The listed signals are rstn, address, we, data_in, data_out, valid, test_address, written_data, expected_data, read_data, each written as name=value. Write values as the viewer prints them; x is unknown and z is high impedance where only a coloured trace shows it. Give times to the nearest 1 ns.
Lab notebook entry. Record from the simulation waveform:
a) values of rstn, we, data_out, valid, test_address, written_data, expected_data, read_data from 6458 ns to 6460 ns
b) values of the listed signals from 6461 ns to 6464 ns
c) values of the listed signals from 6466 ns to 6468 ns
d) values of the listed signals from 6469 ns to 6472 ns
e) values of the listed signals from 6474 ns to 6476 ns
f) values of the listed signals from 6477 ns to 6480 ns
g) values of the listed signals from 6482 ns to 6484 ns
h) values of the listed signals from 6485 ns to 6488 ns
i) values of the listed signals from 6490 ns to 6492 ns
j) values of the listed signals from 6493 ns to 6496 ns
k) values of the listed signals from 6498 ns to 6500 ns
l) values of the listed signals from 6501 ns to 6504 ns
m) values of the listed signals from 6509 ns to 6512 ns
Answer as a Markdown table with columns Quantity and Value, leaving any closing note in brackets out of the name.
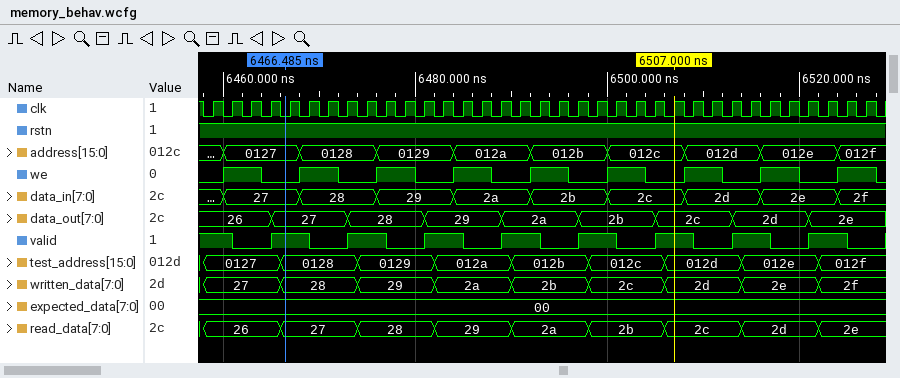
| Quantity | Value |
|---|---|
| values of rstn, we, data_out, valid, test_address, written_data, expected_data, read_data from 6458 ns to 6460 ns | rstn=1, we=0, data_out=26, valid=1, test_address=0127, written_data=27, expected_data=00, read_data=26 |
| values of the listed signals from 6461 ns to 6464 ns | rstn=1, address=0127, we=1, data_in=27, data_out=26, valid=0, test_address=0127, written_data=27, expected_data=00, read_data=26 |
| values of the listed signals from 6466 ns to 6468 ns | rstn=1, address=0127, we=0, data_in=27, data_out=27, valid=1, test_address=0128, written_data=28, expected_data=00, read_data=27 |
| values of the listed signals from 6469 ns to 6472 ns | rstn=1, address=0128, we=1, data_in=28, data_out=27, valid=0, test_address=0128, written_data=28, expected_data=00, read_data=27 |
| values of the listed signals from 6474 ns to 6476 ns | rstn=1, address=0128, we=0, data_in=28, data_out=28, valid=1, test_address=0129, written_data=29, expected_data=00, read_data=28 |
| values of the listed signals from 6477 ns to 6480 ns | rstn=1, address=0129, we=1, data_in=29, data_out=28, valid=0, test_address=0129, written_data=29, expected_data=00, read_data=28 |
| values of the listed signals from 6482 ns to 6484 ns | rstn=1, address=0129, we=0, data_in=29, data_out=29, valid=1, test_address=012a, written_data=2a, expected_data=00, read_data=29 |
| values of the listed signals from 6485 ns to 6488 ns | rstn=1, address=012a, we=1, data_in=2a, data_out=29, valid=0, test_address=012a, written_data=2a, expected_data=00, read_data=29 |
| values of the listed signals from 6490 ns to 6492 ns | rstn=1, address=012a, we=0, data_in=2a, data_out=2a, valid=1, test_address=012b, written_data=2b, expected_data=00, read_data=2a |
| values of the listed signals from 6493 ns to 6496 ns | rstn=1, address=012b, we=1, data_in=2b, data_out=2a, valid=0, test_address=012b, written_data=2b, expected_data=00, read_data=2a |
| values of the listed signals from 6498 ns to 6500 ns | rstn=1, address=012b, we=0, data_in=2b, data_out=2b, valid=1, test_address=012c, written_data=2c, expected_data=00, read_data=2b |
| values of the listed signals from 6501 ns to 6504 ns | rstn=1, address=012c, we=1, data_in=2c, data_out=2b, valid=0, test_address=012c, written_data=2c, expected_data=00, read_data=2b |
| values of the listed signals from 6509 ns to 6512 ns | rstn=1, address=012d, we=1, data_in=2d, data_out=2c, valid=0, test_address=012d, written_data=2d, expected_data=00, read_data=2c |
